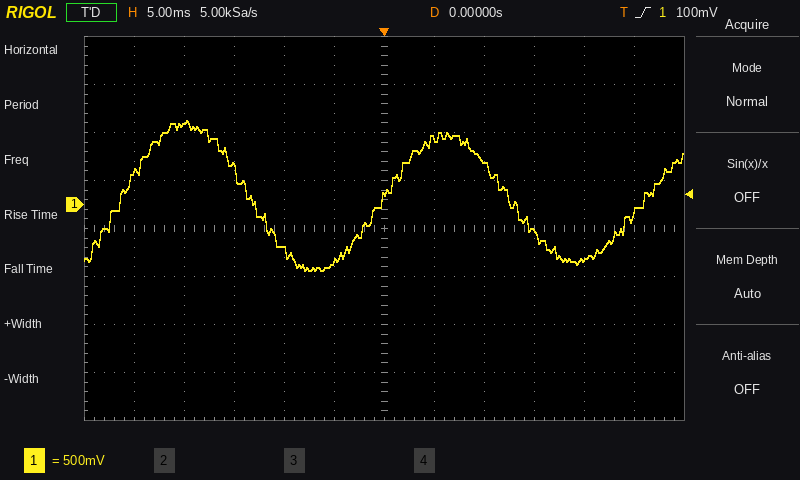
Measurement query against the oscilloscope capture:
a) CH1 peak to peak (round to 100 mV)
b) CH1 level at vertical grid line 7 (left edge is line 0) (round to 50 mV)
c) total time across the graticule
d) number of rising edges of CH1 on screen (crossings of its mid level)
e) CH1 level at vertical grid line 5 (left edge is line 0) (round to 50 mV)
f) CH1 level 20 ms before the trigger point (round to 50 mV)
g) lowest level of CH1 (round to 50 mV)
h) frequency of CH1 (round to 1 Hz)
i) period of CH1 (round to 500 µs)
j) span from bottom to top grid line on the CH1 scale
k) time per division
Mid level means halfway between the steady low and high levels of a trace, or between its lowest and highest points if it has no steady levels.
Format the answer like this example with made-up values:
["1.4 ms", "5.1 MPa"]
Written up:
["1.60 V", "700 mV", "60 ms", "3", "-600 mV", "850 mV", "-700 mV", "38 Hz", "26.0 ms", "4 V", "5 ms"]
